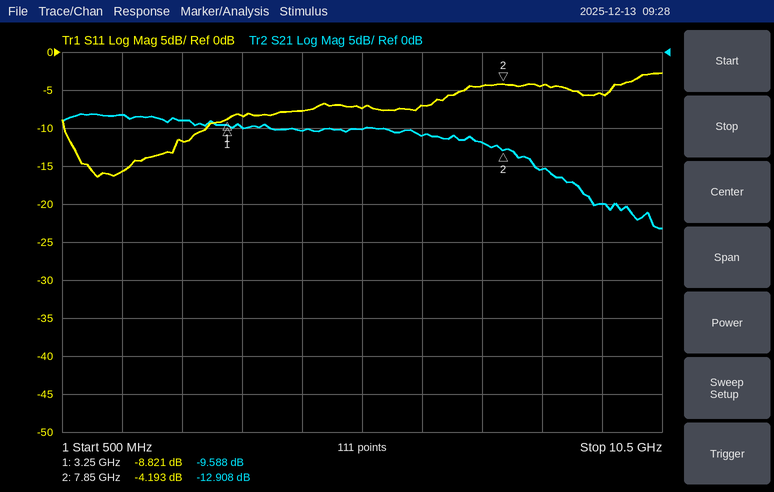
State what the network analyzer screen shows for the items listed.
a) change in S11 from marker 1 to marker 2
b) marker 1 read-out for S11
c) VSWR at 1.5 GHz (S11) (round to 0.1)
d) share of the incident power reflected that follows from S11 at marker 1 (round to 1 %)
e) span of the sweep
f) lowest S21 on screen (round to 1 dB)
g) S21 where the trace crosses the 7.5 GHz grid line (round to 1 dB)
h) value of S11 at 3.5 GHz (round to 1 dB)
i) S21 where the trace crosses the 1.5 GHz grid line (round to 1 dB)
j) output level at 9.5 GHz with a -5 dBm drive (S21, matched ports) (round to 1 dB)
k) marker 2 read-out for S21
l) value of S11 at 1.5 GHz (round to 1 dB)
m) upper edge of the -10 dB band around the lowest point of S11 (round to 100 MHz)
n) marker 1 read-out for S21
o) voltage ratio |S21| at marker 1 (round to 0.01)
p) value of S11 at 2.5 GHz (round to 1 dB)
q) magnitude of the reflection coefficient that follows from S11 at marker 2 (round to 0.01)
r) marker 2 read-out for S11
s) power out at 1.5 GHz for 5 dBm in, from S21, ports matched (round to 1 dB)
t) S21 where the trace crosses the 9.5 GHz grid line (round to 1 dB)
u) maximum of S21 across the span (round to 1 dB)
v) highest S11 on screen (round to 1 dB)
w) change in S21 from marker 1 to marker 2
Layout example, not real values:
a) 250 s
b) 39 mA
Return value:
a) 4.628 dB
b) -8.821 dB
c) 1.4
d) 13 %
e) 10 GHz
f) -23 dB
g) -12 dB
h) -8 dB
i) -8 dB
j) -25 dBm
k) -12.908 dB
l) -16 dB
m) 2.9 GHz
n) -9.588 dB
o) 0.33
p) -12 dB
q) 0.62
r) -4.193 dB
s) -3 dBm
t) -20 dB
u) -8 dB
v) -3 dB
w) -3.320 dB
